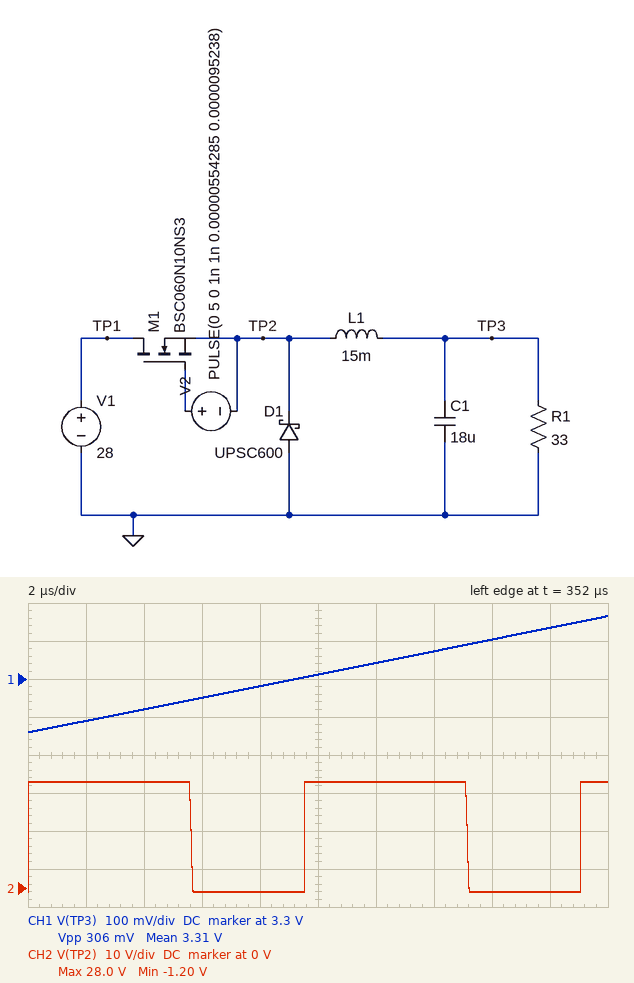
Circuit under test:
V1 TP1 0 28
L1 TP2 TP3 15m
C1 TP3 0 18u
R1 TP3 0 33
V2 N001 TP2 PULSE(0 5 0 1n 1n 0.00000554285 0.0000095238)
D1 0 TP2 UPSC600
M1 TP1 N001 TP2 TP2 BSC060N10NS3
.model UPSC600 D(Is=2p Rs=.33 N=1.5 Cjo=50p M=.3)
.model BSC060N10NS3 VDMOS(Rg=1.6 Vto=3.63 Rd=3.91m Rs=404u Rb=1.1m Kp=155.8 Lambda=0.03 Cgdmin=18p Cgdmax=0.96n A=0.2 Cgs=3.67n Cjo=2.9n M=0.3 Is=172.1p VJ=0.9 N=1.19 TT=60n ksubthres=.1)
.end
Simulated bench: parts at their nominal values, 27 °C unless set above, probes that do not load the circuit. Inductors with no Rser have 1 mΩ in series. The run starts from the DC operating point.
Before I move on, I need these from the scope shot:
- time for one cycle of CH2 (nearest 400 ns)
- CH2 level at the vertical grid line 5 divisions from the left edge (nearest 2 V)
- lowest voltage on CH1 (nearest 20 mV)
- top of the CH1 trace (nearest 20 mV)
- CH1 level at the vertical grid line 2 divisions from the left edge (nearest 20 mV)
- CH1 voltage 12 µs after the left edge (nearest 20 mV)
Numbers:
9.6 µs
28 V
3.16 V
3.46 V
3.22 V
3.34 V
